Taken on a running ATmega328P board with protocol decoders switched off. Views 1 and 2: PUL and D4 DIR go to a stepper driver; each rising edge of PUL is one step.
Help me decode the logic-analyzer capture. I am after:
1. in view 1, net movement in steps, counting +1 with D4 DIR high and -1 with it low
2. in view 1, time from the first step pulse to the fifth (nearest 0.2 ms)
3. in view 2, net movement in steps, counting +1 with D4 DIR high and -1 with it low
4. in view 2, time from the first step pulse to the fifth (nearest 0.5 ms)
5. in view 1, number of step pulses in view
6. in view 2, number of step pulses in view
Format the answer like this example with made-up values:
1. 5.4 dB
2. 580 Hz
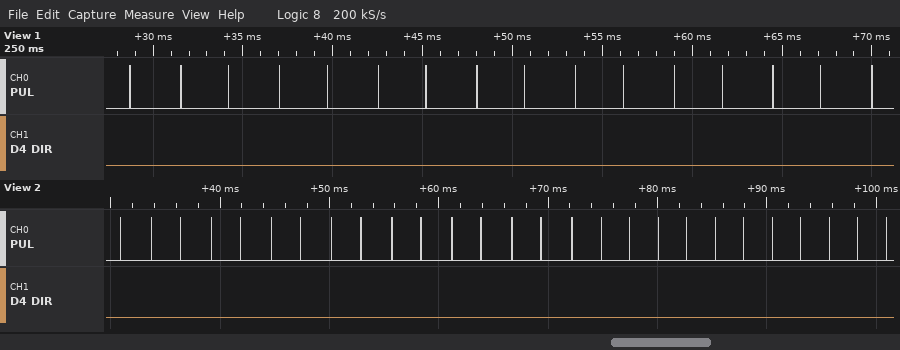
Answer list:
1. -16
2. 11.0 ms
3. -27
4. 11.0 ms
5. 16
6. 27
